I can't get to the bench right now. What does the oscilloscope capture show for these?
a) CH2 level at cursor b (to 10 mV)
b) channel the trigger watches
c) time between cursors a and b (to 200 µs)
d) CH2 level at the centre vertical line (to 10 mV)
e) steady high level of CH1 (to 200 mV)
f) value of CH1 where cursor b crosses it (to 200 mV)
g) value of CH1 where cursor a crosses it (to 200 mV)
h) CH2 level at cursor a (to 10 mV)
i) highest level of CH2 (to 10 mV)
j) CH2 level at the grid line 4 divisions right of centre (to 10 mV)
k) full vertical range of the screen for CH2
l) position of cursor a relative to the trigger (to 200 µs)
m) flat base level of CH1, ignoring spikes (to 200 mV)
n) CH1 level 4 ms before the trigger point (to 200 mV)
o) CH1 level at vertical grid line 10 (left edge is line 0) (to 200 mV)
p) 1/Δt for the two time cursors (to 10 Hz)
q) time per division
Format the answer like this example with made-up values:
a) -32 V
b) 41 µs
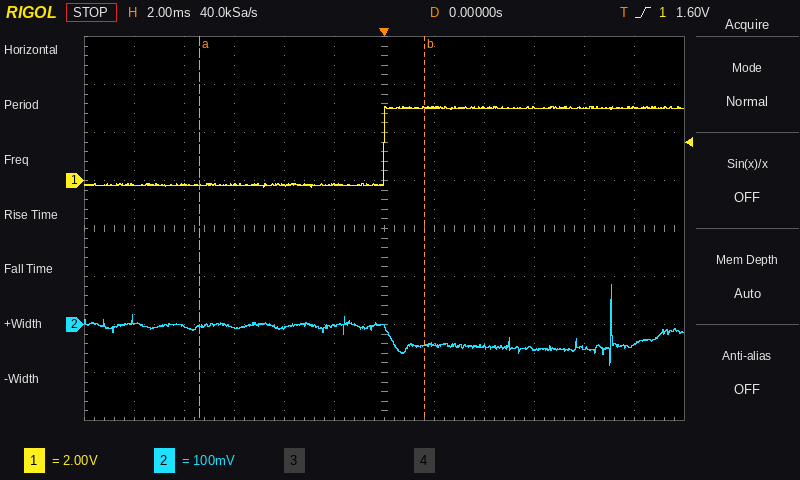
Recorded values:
a) -40 mV
b) CH1
c) 9.0 ms
d) -10 mV
e) 3.0 V
f) 3.0 V
g) -200 mV
h) 0 mV
i) 80 mV
j) -50 mV
k) 800 mV
l) -7.4 ms
m) -200 mV
n) -200 mV
o) 3.0 V
p) 110 Hz
q) 2 ms
